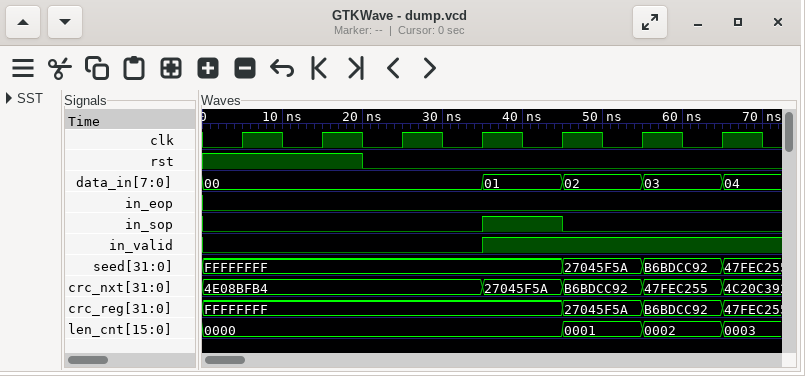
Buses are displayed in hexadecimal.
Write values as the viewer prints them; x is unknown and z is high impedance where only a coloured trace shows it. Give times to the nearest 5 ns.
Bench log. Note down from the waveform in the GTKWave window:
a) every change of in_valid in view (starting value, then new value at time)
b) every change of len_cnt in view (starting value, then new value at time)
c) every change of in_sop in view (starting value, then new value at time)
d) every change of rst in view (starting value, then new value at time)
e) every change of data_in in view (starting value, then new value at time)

0, 1 at 35 ns
0000, 0001 at 45 ns, 0002 at 55 ns, 0003 at 65 ns
0, 1 at 35 ns, 0 at 45 ns
1, 0 at 20 ns
00, 01 at 35 ns, 02 at 45 ns, 03 at 55 ns, 04 at 65 ns
